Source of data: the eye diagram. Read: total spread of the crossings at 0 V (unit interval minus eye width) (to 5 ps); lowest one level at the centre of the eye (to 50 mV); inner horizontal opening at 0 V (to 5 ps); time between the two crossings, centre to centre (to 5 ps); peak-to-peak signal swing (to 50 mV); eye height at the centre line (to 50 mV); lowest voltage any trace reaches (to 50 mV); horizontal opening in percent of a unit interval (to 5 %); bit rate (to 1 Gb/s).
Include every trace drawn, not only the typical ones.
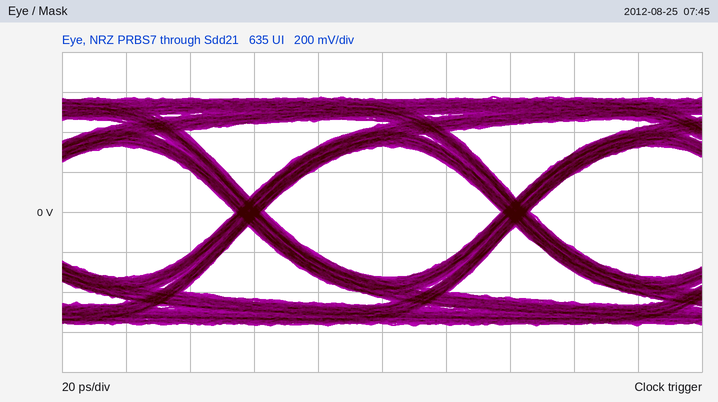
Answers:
10 ps
350 mV
75 ps
85 ps
1.15 V
650 mV
-550 mV
90 %
12 Gb/s
